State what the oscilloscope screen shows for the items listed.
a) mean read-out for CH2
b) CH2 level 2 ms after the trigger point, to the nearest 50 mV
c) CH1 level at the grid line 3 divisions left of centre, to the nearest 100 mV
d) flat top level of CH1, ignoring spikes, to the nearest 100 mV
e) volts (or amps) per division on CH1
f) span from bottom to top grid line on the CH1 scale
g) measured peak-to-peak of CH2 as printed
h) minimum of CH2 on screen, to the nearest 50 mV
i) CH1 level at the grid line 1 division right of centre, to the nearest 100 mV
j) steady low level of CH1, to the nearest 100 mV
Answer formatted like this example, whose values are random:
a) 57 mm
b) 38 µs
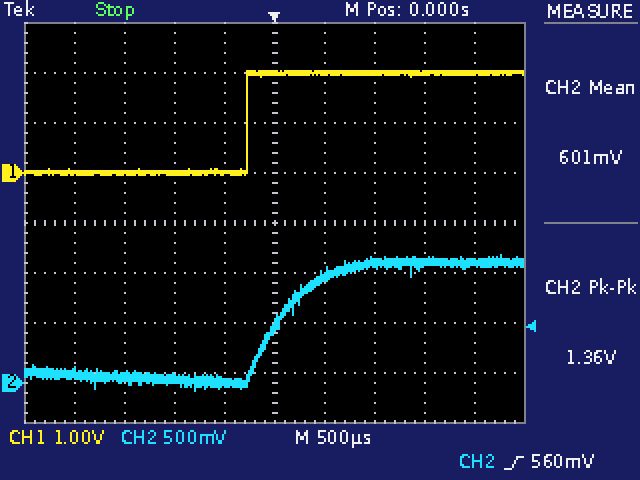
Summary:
a) 601 mV
b) 1.20 V
c) 0.0 V
d) 2.0 V
e) 1 V
f) 8 V
g) 1.36 V
h) -100 mV
i) 2.0 V
j) 0.0 V
